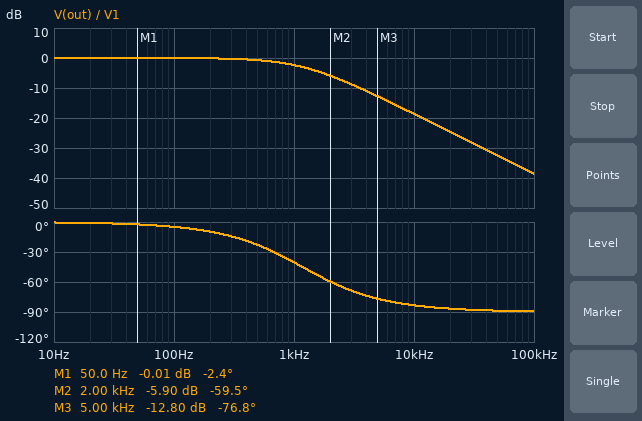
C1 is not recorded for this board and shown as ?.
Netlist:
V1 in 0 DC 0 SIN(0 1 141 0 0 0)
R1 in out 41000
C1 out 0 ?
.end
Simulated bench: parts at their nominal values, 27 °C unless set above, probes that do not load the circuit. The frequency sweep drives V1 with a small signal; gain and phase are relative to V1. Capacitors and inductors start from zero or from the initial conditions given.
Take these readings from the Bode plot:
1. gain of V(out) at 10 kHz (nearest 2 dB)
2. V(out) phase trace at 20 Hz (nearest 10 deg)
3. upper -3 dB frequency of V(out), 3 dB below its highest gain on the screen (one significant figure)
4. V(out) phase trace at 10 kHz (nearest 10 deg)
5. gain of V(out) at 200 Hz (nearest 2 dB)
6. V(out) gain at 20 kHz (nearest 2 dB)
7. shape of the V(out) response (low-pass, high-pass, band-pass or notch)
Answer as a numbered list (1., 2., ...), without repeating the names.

1. -18 dB
2. 0 deg
3. 1 kHz
4. -80 deg
5. 0 dB
6. -24 dB
7. low-pass
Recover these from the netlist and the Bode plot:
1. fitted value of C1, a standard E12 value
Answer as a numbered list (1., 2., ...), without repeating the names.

1. 3.3 nF
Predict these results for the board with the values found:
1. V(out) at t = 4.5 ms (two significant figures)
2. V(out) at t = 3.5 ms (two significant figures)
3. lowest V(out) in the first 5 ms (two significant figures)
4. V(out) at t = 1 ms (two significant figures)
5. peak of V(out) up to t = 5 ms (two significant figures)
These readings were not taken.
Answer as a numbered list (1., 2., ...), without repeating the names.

1. -660 mV
2. 160 mV
3. -910 mV
4. 690 mV
5. 990 mV
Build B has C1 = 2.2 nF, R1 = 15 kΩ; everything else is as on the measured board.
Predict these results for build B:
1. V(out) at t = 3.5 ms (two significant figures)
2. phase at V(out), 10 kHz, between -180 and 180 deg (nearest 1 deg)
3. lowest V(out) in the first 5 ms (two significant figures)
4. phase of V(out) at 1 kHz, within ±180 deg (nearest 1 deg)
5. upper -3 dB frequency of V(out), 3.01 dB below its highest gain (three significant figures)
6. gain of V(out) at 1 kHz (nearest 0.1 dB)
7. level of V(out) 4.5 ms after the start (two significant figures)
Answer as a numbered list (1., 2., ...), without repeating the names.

1. 70 mV
2. -64 deg
3. -950 mV
4. -12 deg
5. 4.82 kHz
6. -0.2 dB
7. -730 mV
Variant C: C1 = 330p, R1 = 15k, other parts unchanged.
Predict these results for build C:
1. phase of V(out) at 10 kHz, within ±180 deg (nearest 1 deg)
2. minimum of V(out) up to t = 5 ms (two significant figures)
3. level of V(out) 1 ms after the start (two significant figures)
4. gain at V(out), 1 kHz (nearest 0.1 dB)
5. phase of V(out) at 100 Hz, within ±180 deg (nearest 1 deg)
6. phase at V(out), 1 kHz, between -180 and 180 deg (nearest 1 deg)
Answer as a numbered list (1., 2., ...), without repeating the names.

1. -17 deg
2. -960 mV
3. 770 mV
4. 0 dB
5. 0 deg
6. -2 deg
